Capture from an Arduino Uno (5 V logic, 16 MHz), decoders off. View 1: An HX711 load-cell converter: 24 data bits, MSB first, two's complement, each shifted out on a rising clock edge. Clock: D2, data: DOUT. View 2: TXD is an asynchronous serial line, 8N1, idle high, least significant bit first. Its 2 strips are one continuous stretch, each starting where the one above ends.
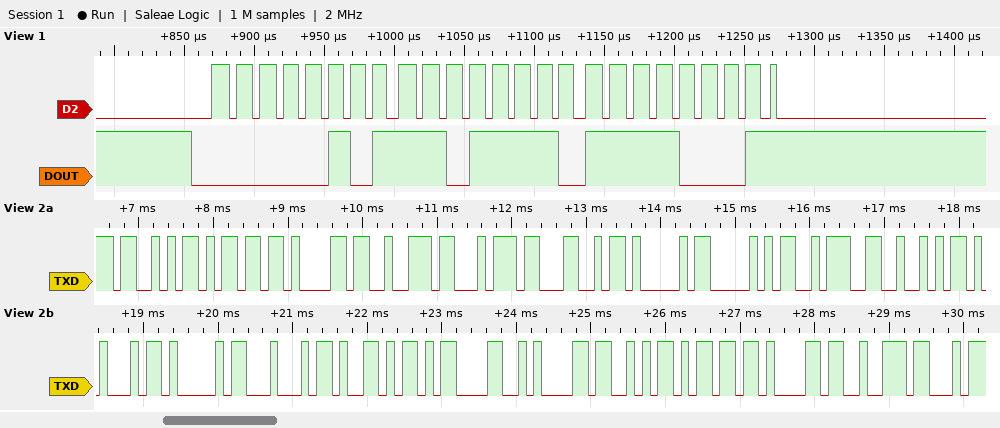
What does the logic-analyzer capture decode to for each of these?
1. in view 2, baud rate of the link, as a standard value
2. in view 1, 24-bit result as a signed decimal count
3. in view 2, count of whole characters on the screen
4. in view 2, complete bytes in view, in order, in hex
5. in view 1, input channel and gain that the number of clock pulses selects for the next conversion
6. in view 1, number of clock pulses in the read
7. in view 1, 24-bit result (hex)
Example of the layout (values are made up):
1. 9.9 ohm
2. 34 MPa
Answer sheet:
1. 9600 baud
2. 384753
3. 20
4. 53 6D 61 72 74 4C 41 50 3A 52 45 41 44 59 0D 0A 53 6D 61 72
5. channel A, gain 128
6. 25
7. 0x05DEF1
